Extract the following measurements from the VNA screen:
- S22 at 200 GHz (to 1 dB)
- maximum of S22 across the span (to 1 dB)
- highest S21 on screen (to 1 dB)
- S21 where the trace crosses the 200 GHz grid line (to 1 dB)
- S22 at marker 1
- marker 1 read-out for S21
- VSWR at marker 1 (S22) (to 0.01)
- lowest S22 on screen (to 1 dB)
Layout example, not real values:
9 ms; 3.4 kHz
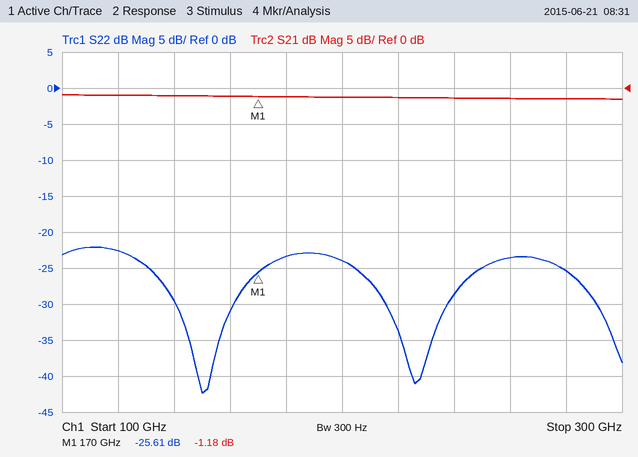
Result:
-24 dB; -22 dB; -1 dB; -1 dB; -25.61 dB; -1.18 dB; 1.11; -42 dB
